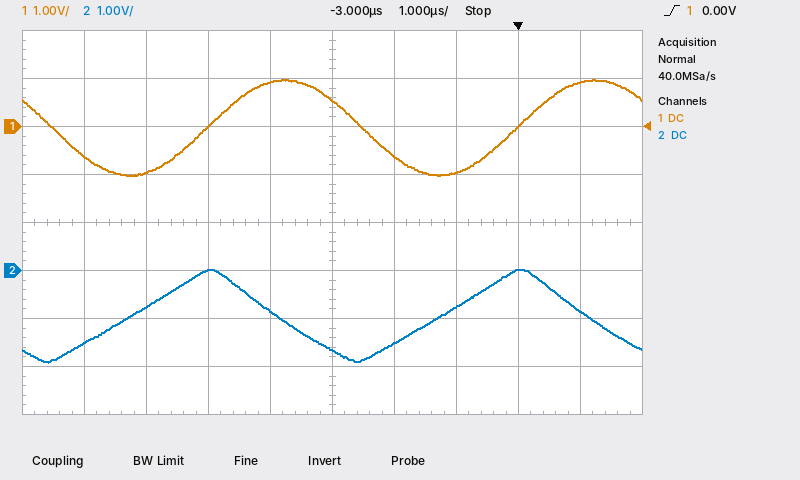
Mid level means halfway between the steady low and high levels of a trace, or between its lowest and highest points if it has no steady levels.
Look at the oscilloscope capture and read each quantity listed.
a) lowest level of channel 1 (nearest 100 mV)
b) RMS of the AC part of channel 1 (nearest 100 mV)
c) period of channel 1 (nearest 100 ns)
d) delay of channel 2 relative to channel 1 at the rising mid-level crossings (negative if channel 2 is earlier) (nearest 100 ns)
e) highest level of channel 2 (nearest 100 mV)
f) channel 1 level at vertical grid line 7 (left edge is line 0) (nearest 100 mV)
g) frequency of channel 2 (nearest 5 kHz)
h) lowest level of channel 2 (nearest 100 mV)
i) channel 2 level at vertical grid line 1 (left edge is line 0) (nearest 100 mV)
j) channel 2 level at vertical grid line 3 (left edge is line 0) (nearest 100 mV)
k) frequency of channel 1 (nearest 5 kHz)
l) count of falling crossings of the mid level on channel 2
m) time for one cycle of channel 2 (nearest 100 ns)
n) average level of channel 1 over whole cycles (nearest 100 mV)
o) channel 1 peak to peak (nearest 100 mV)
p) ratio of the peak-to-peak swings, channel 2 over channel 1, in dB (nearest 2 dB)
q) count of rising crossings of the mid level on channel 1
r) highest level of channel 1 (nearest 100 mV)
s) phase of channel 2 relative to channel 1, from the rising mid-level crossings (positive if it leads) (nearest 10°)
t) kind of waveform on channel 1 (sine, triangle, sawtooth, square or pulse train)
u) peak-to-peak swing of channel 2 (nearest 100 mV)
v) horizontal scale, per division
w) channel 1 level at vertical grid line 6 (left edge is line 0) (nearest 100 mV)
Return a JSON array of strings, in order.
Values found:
["-1.0 V", "700 mV", "5.0 µs", "-1.2 µs", "0.0 V", "-1.0 V", "200 kHz", "-1.9 V", "-1.5 V", "0.0 V", "200 kHz", "2", "5.0 µs", "0.0 V", "2.0 V", "0 dB", "2", "1.0 V", "+90°", "sine", "1.9 V", "1 µs", "-600 mV"]
